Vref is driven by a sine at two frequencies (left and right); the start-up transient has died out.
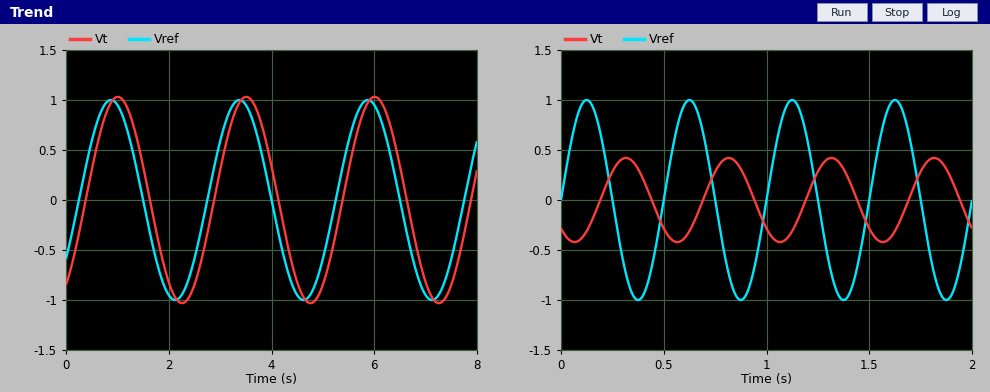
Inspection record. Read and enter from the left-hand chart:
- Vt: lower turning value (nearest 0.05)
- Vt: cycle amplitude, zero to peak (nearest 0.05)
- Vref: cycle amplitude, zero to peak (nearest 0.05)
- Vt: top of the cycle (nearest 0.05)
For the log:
-1.05
1.05
1.00
1.05
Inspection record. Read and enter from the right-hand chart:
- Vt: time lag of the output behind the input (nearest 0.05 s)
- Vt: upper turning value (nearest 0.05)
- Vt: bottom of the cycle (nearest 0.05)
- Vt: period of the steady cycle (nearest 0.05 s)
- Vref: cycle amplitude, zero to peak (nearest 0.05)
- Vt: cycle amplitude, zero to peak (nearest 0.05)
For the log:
0.20 s
0.40
-0.40
0.50 s
1.00
0.40
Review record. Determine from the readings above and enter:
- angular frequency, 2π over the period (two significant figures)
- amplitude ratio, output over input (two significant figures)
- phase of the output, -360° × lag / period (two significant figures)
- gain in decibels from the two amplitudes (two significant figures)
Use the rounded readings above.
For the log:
13 rad/s
0.40
-140°
-8.0 dB
